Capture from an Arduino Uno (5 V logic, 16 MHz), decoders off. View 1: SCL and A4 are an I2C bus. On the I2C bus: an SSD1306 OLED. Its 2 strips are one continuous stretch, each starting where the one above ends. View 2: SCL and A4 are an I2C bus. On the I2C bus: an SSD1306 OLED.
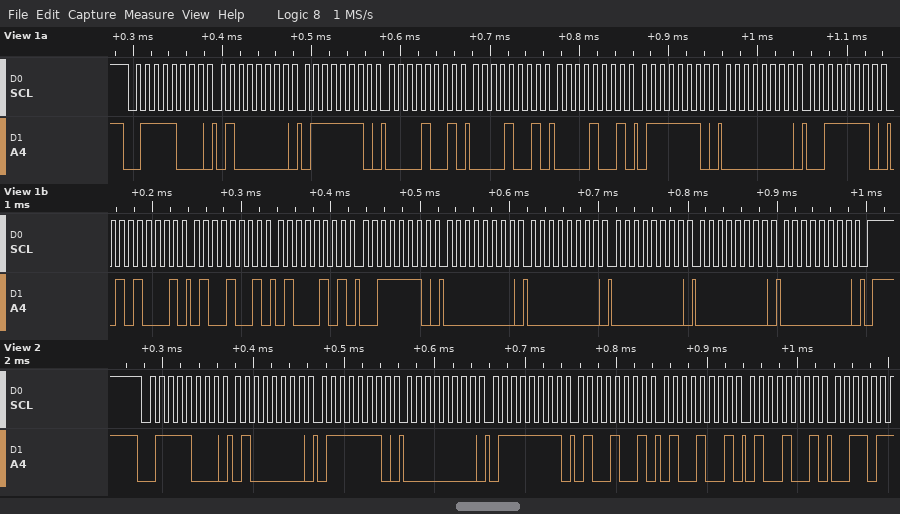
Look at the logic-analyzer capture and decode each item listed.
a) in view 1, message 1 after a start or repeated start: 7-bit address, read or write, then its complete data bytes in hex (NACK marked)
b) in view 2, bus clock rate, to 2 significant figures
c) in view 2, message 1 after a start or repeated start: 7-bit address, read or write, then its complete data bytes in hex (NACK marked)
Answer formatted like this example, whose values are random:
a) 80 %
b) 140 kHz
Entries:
a) 0x3C write: 40 7E 09 09 09 7E 00 3E 51 49 45 3E 00 00 00 00 00
b) 100 kHz
c) 0x3C write: 40 7E 00 7F 49 49 49
